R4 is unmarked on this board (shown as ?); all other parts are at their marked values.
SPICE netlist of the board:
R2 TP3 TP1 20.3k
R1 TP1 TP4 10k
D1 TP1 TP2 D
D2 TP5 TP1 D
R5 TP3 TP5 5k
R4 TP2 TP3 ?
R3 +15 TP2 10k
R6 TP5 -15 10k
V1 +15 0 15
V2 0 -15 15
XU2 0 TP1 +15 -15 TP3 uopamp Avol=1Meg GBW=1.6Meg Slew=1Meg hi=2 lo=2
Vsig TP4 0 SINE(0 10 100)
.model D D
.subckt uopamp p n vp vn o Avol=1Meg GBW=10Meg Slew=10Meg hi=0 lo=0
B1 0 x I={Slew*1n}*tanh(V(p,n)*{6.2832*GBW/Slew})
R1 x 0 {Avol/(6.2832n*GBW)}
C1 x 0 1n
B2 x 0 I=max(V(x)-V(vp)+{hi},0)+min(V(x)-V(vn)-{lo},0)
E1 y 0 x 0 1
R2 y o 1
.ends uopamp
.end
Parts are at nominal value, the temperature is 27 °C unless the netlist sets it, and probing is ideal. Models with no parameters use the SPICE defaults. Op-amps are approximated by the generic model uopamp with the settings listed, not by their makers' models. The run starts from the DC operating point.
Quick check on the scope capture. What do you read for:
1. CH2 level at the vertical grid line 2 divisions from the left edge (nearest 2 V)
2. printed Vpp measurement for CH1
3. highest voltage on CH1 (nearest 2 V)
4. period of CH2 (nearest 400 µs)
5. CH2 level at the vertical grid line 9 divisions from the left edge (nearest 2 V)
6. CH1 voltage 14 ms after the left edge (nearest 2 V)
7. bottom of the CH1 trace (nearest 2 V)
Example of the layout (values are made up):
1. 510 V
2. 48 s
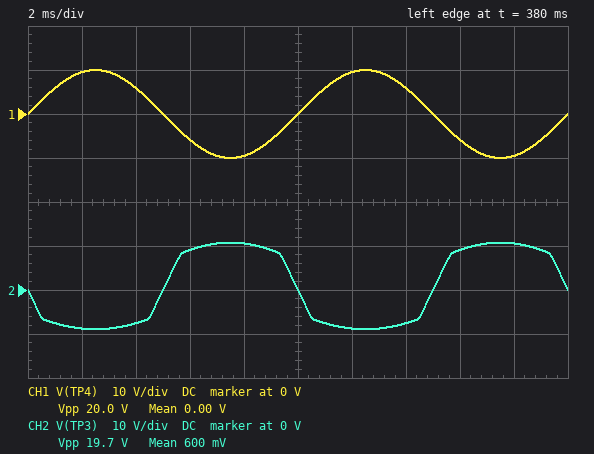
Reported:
1. -8 V
2. 20.0 V
3. 10 V
4. 10.0 ms
5. 10 V
6. 6 V
7. -10 V
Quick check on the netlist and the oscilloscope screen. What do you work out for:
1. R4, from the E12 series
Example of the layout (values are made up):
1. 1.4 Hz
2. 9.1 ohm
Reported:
1. 3.9 kΩ
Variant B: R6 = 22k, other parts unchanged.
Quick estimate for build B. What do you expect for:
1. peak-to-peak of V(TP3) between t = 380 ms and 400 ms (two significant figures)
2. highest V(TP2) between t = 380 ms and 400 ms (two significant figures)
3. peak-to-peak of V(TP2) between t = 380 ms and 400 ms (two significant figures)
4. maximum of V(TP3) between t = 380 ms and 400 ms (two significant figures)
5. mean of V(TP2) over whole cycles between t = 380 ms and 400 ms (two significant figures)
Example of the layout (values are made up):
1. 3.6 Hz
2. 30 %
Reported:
1. 16 V
2. 9.5 V
3. 10 V
4. 7.4 V
5. 4.1 V
